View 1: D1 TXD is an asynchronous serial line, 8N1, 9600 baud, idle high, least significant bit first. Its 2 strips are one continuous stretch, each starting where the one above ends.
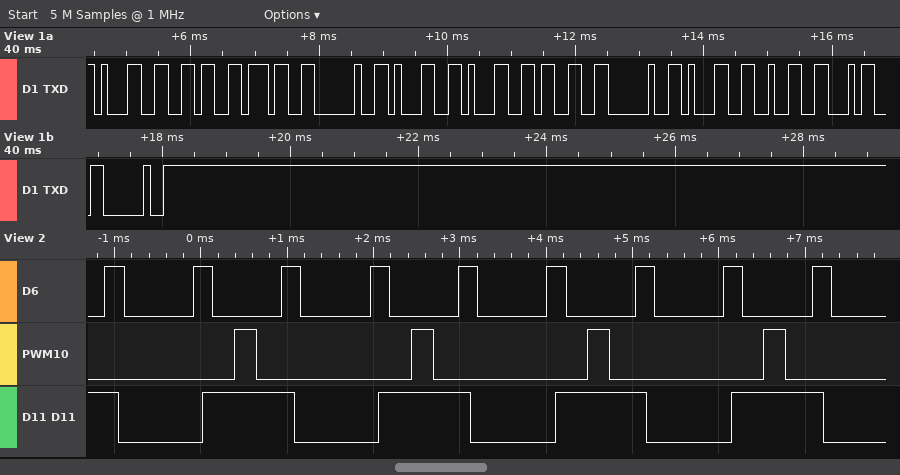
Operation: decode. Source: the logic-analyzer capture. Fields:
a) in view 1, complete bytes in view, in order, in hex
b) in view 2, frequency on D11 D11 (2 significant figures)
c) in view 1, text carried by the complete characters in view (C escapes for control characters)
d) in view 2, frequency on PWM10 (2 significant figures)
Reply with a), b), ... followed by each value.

a) 31 36 37 20 31 31 33 20 31 32 34 20
b) 490 Hz
c) "167 113 124 "
d) 490 Hz
